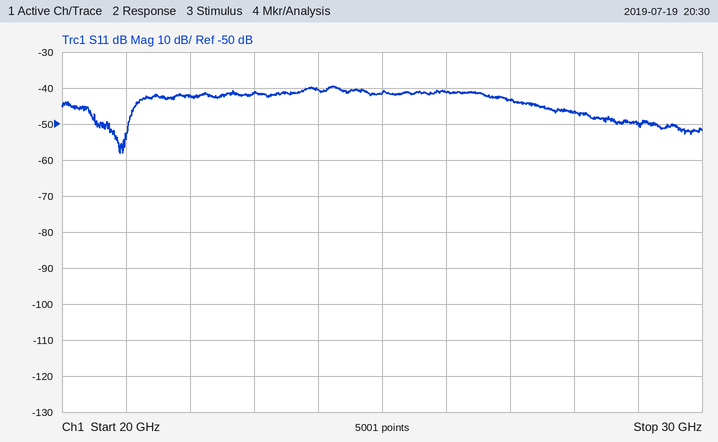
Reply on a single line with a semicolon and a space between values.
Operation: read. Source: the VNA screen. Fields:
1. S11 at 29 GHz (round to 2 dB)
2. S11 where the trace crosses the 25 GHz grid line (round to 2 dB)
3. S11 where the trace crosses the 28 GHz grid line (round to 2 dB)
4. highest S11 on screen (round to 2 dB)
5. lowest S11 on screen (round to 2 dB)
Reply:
-50 dB; -42 dB; -46 dB; -40 dB; -58 dB
